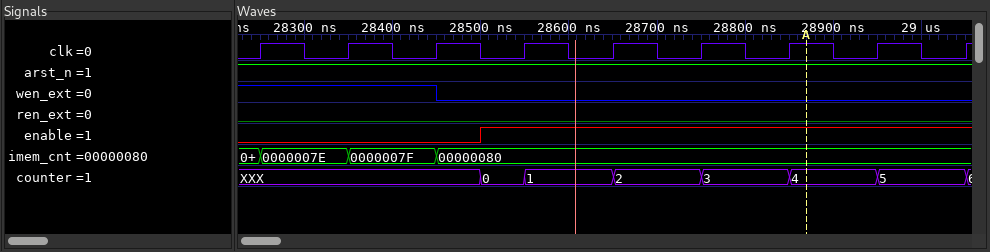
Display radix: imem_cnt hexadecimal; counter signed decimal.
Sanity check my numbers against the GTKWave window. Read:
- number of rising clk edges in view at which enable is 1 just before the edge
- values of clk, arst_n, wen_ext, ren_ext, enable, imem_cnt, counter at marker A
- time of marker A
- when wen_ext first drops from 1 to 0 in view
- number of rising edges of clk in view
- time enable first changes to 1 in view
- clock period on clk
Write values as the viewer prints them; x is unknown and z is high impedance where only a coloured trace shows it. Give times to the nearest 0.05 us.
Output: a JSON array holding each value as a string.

["6", "clk=1, arst_n=1, wen_ext=0, ren_ext=0, enable=1, imem_cnt=00000080, counter=4", "28.85 us", "28.45 us", "9", "28.5 us", "0.1 us"]
